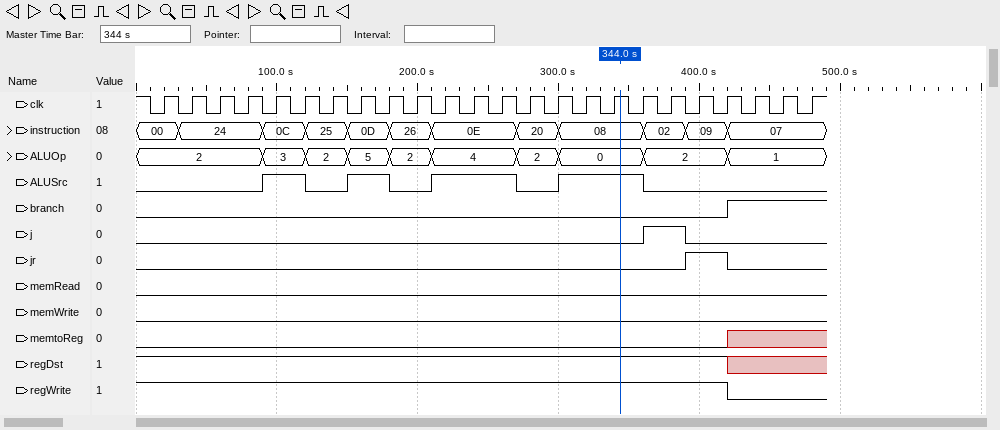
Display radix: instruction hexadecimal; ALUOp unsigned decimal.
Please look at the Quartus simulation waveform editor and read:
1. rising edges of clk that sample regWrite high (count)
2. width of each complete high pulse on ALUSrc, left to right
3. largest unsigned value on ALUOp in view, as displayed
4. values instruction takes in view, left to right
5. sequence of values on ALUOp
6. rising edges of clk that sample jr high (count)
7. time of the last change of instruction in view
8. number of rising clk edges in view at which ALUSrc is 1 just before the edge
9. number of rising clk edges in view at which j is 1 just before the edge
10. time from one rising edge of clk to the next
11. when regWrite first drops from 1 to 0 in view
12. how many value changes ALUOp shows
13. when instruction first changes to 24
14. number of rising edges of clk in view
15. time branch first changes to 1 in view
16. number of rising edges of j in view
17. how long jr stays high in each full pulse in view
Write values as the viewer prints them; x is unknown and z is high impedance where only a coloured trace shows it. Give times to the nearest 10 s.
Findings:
21
30 s, 30 s, 60 s, 60 s
5
00, 24, 0C, 25, 0D, 26, 0E, 20, 08, 02, 09, 07
2, 3, 2, 5, 2, 4, 2, 0, 2, 1
2
420 s
10
1
20 s
420 s
9
30 s
24
420 s
1
30 s
